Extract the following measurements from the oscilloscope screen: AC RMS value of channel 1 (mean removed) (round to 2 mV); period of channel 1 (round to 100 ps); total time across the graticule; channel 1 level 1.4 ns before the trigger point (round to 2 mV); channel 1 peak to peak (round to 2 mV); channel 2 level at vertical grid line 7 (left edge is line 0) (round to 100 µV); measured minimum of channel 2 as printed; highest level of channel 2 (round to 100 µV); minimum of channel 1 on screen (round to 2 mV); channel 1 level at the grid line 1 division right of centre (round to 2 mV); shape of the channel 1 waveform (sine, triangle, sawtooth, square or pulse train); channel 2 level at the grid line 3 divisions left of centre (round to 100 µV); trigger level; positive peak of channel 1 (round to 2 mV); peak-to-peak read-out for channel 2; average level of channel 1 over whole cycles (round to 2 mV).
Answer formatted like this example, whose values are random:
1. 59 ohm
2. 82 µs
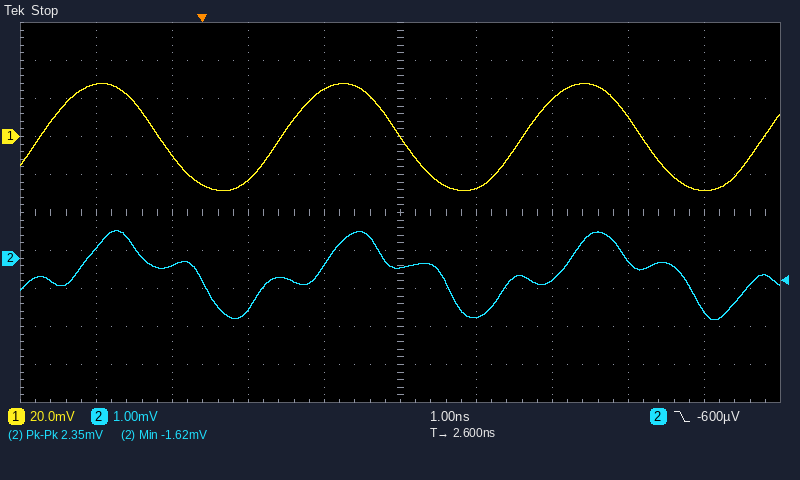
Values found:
1. 20 mV
2. 3.2 ns
3. 10 ns
4. 28 mV
5. 56 mV
6. -600 µV
7. -1.62 mV
8. 700 µV
9. -28 mV
10. -28 mV
11. sine
12. -200 µV
13. -600 µV
14. 28 mV
15. 2.35 mV
16. 0 mV
